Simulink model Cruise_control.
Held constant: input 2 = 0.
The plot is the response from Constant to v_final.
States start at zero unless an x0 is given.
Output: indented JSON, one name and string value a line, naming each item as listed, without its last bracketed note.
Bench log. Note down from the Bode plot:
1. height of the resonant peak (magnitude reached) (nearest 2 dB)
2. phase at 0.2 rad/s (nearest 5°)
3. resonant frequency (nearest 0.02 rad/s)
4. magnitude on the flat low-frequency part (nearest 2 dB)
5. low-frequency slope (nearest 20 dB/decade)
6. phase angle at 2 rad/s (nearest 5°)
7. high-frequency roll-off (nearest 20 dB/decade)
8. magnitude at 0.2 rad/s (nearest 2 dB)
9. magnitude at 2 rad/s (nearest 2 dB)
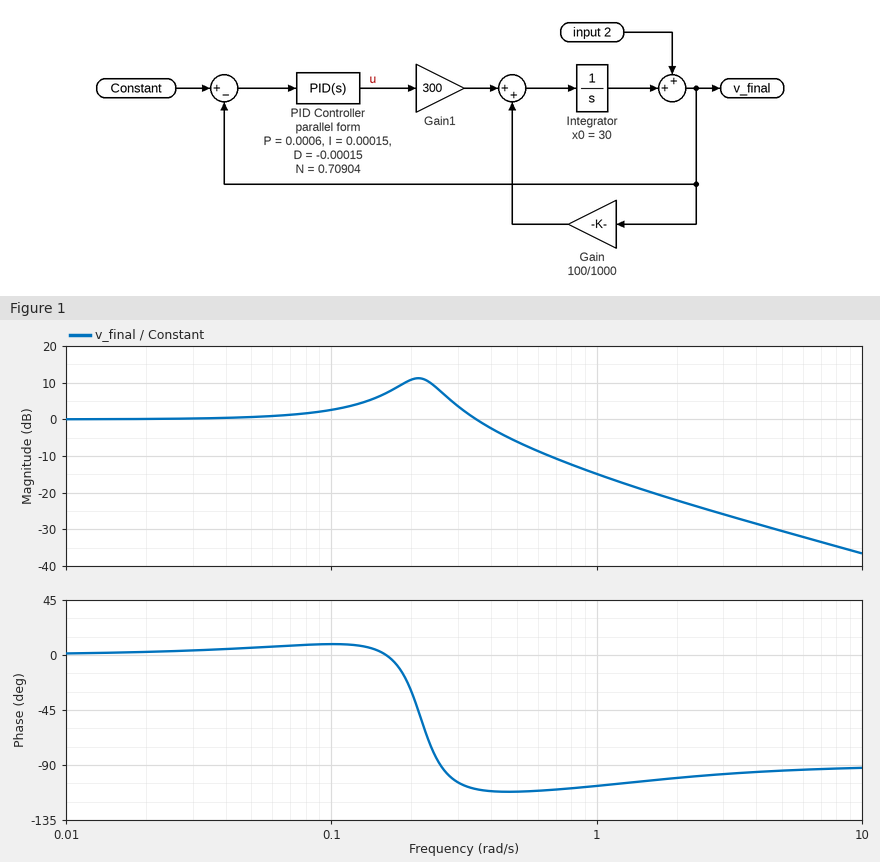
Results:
{
  "height of the resonant peak (magnitude reached)": "12 dB",
  "phase at 0.2 rad/s": "-30°",
  "resonant frequency": "0.22 rad/s",
  "magnitude on the flat low-frequency part": "0 dB",
  "low-frequency slope": "0 dB/decade",
  "phase angle at 2 rad/s": "-100°",
  "high-frequency roll-off": "-20 dB/decade",
  "magnitude at 0.2 rad/s": "10 dB",
  "magnitude at 2 rad/s": "-22 dB"
}
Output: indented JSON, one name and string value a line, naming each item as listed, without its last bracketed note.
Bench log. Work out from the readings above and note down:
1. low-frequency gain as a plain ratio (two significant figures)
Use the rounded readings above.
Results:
{
  "low-frequency gain as a plain ratio": "1.0"
}
